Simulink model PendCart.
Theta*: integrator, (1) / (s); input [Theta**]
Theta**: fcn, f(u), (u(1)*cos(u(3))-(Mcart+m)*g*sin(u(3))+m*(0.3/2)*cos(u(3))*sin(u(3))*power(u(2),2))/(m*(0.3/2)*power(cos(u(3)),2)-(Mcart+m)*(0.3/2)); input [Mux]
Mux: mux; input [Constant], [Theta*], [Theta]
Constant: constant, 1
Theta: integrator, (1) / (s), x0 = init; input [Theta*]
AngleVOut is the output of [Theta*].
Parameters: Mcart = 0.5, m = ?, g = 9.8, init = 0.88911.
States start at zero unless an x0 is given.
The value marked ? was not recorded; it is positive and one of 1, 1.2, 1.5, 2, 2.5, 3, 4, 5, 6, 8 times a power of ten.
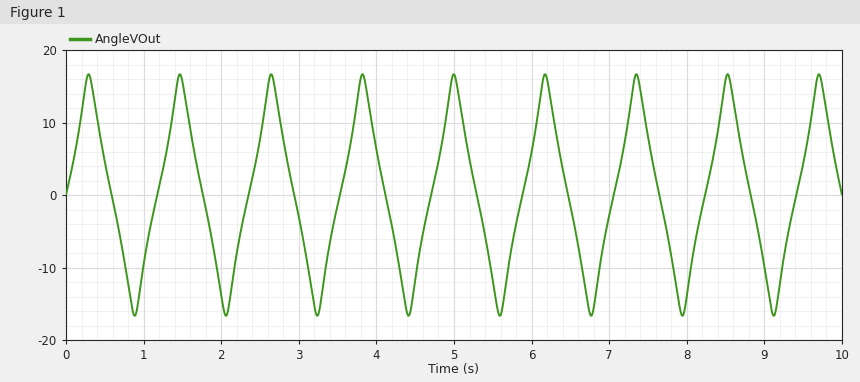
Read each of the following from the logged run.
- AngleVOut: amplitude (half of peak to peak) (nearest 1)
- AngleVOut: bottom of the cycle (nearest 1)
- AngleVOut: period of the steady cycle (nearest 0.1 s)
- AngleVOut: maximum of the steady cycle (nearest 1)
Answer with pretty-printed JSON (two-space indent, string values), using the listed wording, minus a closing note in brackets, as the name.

{
  "AngleVOut: amplitude (half of peak to peak)": "17",
  "AngleVOut: bottom of the cycle": "-17",
  "AngleVOut: period of the steady cycle": "1.2 s",
  "AngleVOut: maximum of the steady cycle": "17"
}
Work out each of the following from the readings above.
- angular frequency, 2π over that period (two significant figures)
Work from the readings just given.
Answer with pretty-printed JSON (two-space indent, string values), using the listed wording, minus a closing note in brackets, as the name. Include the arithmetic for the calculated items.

{
  "angular frequency, 2π over that period": "2π / 1.2 = 5.2 rad/s"
}
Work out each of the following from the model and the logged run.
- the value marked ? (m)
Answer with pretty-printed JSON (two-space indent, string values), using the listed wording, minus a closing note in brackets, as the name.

{
  "the value marked ?": "0.1"
}
